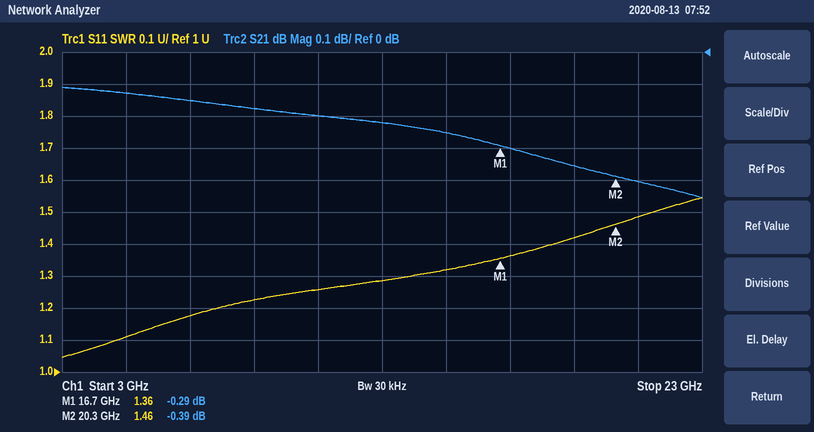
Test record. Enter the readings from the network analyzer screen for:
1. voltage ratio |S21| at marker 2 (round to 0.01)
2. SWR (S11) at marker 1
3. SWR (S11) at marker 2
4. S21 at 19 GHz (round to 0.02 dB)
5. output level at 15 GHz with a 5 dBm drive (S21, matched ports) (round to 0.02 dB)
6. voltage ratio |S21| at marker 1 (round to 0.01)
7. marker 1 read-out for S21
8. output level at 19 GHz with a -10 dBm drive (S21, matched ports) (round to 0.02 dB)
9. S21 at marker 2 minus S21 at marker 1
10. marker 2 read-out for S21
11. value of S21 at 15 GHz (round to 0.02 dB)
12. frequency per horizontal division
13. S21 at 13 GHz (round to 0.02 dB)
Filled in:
0.96
1.36
1.46
-0.36 dB
4.74 dBm
0.97
-0.29 dB
-10.36 dBm
-0.10 dB
-0.39 dB
-0.26 dB
2 GHz
-0.22 dB
